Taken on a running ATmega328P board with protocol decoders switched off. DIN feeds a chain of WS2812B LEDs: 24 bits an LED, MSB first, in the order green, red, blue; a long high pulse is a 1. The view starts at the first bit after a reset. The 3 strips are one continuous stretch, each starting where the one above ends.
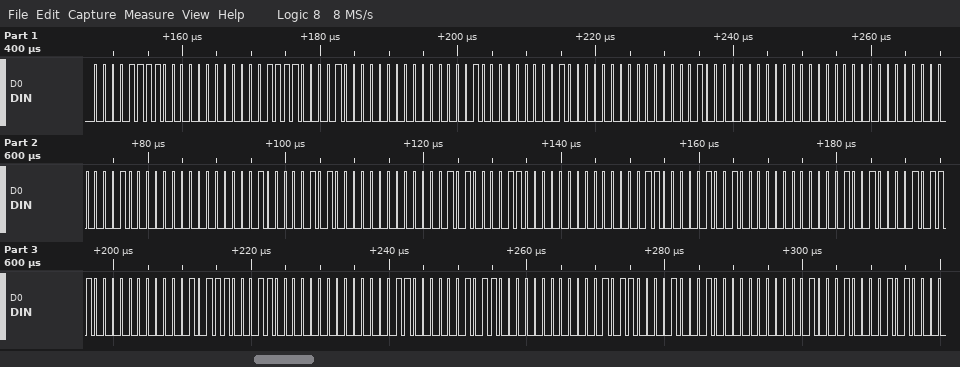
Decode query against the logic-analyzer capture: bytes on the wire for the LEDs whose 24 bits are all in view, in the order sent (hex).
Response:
0F 00 0F 08 00 08 02 00 02 00 00 00 01 00 01 05 00 05 0C 00 0C 12 00 12 17 00 17 18 00 18 16 00 16 11 00 11
